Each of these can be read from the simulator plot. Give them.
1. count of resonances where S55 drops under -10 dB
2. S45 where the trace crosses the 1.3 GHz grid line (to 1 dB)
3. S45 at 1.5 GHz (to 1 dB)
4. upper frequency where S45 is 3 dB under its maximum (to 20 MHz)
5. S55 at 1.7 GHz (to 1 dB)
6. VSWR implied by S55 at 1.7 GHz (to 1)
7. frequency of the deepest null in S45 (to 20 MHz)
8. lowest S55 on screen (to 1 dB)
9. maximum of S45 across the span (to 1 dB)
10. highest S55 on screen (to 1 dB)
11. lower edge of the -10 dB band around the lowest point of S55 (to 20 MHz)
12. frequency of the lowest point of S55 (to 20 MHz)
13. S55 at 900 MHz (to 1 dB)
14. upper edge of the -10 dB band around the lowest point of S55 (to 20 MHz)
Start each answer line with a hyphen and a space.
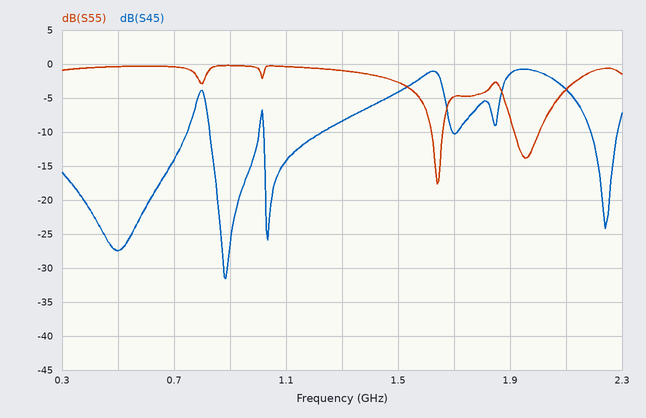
- 2
- -8 dB
- -4 dB
- 2.10 GHz
- -5 dB
- 4
- 880 MHz
- -18 dB
- -1 dB
- 0 dB
- 1.62 GHz
- 1.64 GHz
- 0 dB
- 1.66 GHz
